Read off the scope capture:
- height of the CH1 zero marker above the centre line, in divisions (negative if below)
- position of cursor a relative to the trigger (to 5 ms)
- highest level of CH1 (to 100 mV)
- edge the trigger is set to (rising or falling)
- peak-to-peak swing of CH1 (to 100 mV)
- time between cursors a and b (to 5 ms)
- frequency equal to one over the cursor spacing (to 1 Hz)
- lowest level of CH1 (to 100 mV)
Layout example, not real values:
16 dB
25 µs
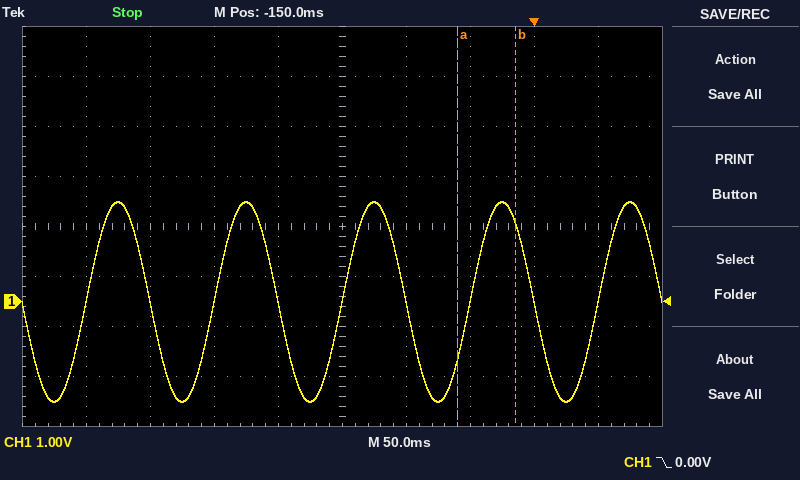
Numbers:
-1.5 div
-60 ms
2.0 V
falling
4.0 V
45 ms
22 Hz
-2.0 V
